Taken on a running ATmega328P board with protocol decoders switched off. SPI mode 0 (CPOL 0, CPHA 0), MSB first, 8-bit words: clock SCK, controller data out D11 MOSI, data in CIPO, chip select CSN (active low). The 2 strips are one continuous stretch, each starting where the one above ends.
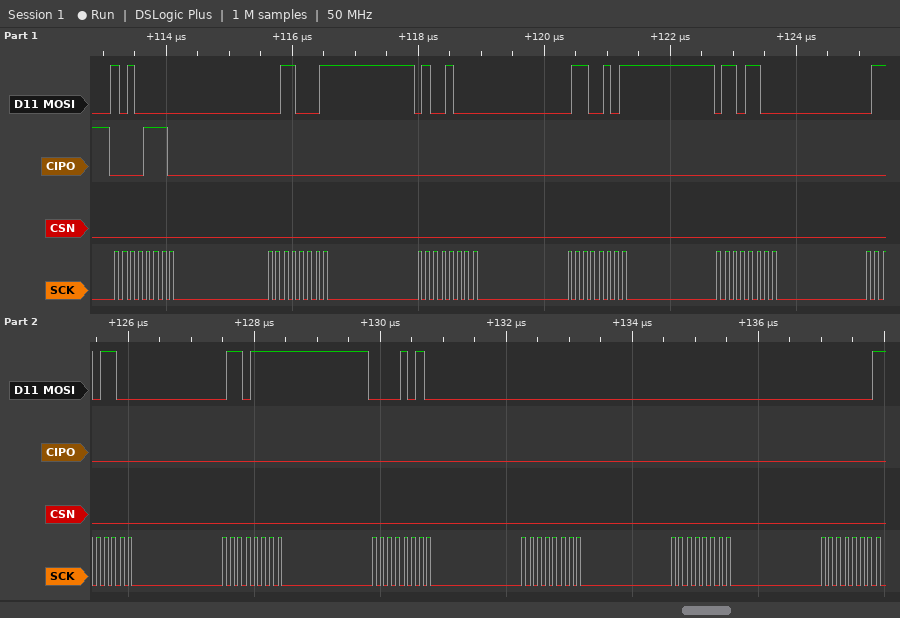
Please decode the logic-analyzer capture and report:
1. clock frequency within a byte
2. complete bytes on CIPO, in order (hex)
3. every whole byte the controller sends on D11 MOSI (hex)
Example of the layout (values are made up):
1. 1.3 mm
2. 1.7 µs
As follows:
1. 8 MHz
2. 0E 00 00 00 00 00 00 00 00 00 00
3. A0 31 48 65 6C 6C 6F 0A 00 00 01
